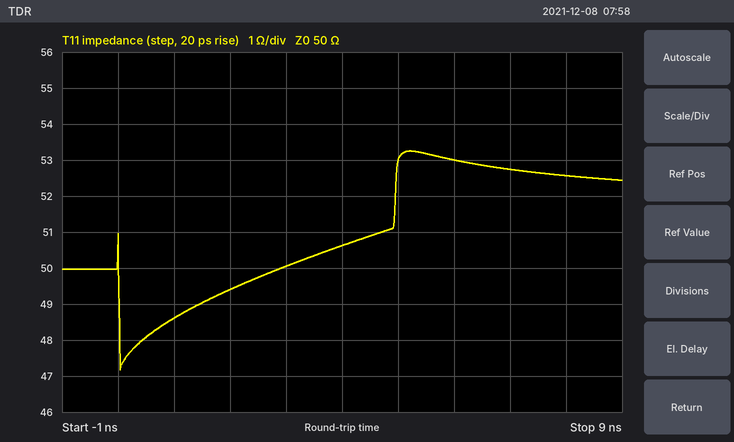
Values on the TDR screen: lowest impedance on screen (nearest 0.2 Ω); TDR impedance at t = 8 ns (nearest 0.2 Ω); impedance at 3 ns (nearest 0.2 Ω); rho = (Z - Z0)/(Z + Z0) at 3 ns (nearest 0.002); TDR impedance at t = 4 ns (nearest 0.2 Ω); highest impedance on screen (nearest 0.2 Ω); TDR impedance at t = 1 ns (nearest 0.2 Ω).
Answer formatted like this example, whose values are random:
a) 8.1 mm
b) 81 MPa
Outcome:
a) 47.2 Ω
b) 52.6 Ω
c) 50.0 Ω
d) 0.000
e) 50.6 Ω
f) 53.2 Ω
g) 48.6 Ω
